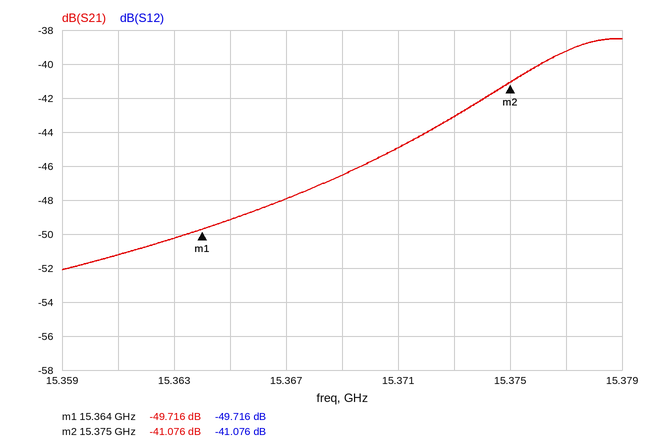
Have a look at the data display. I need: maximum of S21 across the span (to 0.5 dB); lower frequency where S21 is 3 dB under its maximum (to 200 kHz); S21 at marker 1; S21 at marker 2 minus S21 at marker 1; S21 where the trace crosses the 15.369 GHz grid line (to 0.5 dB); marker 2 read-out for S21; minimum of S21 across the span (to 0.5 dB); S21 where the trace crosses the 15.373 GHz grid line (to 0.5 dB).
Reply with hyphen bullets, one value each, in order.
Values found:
- -38.5 dB
- 15.3746 GHz
- -49.716 dB
- 8.640 dB
- -46.5 dB
- -41.076 dB
- -52.0 dB
- -43.0 dB
